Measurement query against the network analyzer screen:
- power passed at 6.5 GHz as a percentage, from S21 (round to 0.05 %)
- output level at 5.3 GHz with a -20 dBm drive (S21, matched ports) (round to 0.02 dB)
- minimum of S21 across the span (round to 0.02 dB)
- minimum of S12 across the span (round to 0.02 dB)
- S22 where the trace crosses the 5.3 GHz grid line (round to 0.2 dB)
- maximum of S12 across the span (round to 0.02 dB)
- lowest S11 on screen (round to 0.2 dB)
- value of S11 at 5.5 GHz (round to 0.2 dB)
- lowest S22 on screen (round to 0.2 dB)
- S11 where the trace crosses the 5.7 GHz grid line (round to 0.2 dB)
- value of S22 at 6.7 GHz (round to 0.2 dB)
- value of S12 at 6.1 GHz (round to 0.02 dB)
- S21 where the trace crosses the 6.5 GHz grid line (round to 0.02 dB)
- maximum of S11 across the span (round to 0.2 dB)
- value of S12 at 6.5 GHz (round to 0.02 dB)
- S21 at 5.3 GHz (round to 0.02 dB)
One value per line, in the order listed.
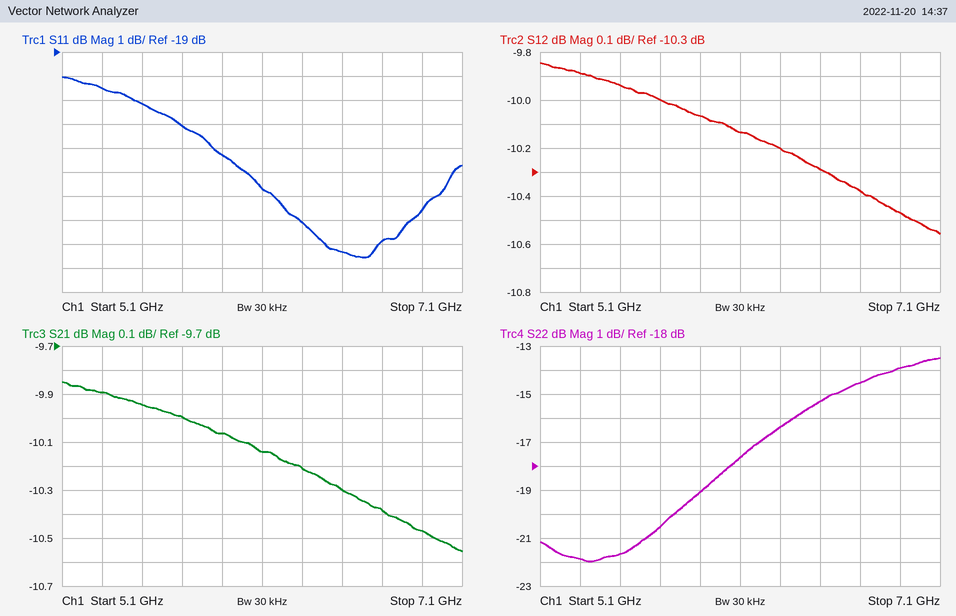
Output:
9.35 %
-29.90 dBm
-10.56 dB
-10.56 dB
-21.8 dB
-9.84 dB
-27.6 dB
-21.2 dB
-22.0 dB
-22.0 dB
-14.6 dB
-10.14 dB
-10.30 dB
-20.0 dB
-10.28 dB
-9.90 dB
